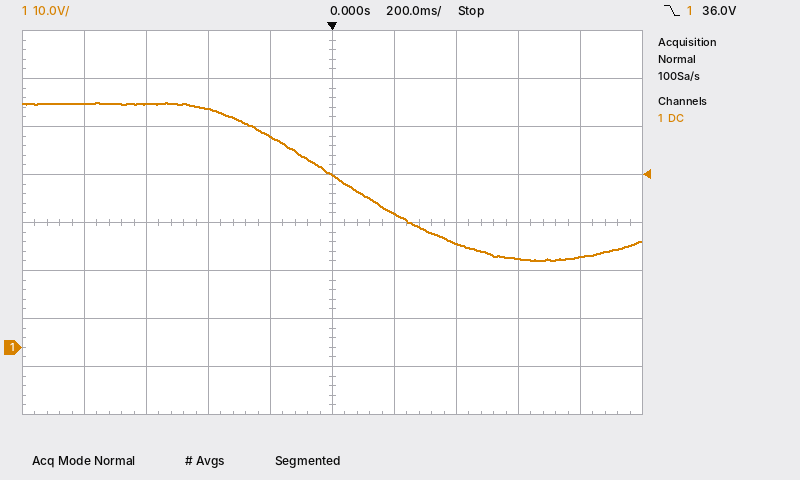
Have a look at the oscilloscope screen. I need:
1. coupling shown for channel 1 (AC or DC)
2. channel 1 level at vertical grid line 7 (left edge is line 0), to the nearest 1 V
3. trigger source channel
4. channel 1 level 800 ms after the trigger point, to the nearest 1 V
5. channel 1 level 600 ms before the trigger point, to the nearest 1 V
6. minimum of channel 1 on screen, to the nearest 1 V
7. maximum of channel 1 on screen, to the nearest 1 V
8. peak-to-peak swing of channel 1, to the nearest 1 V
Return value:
DC
22 V
channel 1
19 V
51 V
18 V
51 V
33 V
